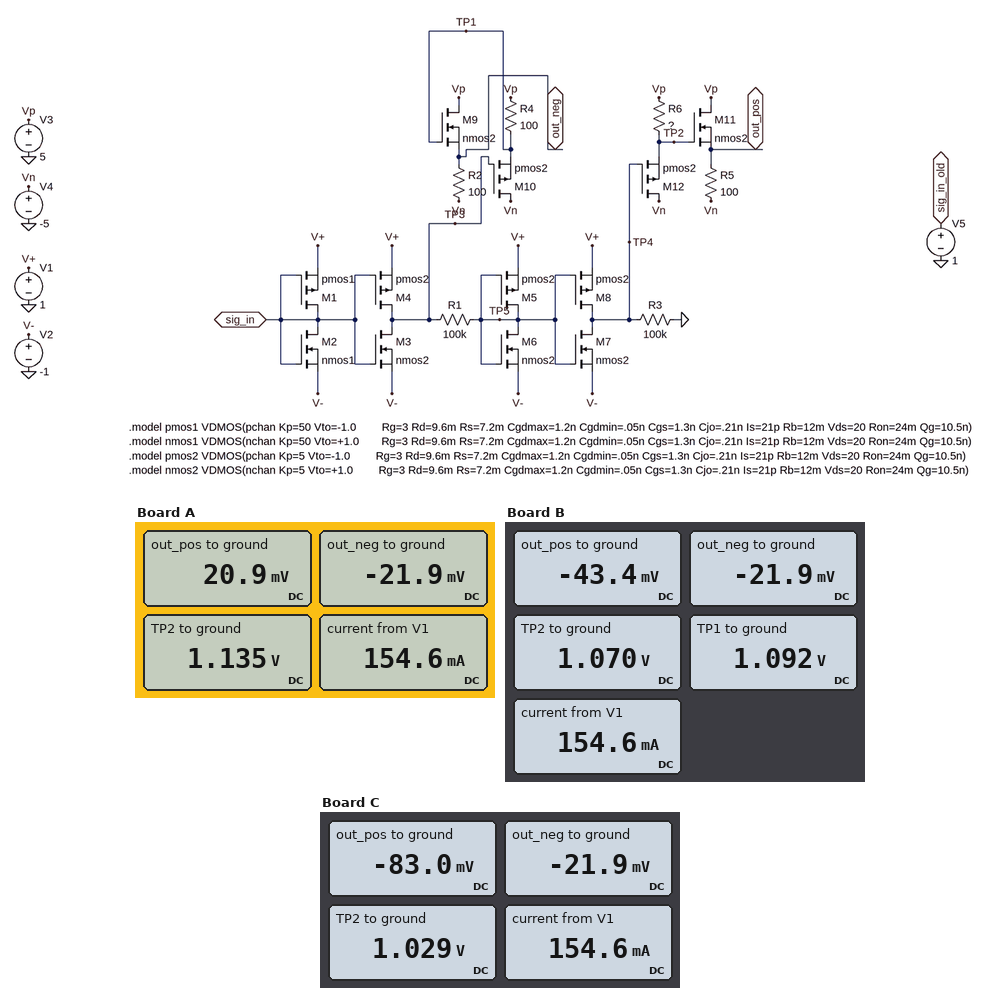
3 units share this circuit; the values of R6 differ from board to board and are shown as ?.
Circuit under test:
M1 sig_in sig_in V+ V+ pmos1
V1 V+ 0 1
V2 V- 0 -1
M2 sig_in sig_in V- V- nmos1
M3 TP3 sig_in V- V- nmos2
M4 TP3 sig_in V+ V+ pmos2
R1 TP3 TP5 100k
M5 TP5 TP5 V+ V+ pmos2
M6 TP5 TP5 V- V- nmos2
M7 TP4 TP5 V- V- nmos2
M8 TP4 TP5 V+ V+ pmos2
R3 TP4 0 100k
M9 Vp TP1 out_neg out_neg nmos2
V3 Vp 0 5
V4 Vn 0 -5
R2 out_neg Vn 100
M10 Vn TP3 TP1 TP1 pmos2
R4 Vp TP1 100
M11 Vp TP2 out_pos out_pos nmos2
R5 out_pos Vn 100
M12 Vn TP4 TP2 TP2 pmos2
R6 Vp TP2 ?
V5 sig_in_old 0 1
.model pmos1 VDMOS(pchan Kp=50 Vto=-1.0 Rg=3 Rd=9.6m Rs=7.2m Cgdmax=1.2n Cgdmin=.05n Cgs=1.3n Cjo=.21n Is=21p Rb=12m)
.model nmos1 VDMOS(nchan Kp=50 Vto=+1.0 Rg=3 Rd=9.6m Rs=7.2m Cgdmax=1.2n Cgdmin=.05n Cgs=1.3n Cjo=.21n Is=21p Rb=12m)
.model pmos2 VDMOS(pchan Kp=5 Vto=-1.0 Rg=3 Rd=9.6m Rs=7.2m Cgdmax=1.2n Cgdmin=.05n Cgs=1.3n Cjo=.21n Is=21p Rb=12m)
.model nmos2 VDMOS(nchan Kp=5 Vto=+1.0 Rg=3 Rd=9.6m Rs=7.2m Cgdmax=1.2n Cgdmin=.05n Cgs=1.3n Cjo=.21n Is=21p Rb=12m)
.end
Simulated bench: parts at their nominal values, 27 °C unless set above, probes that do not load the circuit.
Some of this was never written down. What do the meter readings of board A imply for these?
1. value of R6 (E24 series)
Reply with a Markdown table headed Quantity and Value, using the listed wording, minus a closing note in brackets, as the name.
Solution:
| Quantity | Value |
|---|---|
| value of R6 | 62 Ω |
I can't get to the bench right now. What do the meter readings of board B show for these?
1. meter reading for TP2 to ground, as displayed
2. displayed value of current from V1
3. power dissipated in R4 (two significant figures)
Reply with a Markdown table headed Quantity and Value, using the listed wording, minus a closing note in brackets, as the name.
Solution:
| Quantity | Value |
|---|---|
| meter reading for TP2 to ground, as displayed | 1.070 V |
| displayed value of current from V1 | 154.6 mA |
| power dissipated in R4 | 150 mW |
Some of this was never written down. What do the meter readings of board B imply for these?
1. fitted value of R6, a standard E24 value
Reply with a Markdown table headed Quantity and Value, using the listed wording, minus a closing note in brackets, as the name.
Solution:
| Quantity | Value |
|---|---|
| fitted value of R6, a standard E24 value | 130 Ω |
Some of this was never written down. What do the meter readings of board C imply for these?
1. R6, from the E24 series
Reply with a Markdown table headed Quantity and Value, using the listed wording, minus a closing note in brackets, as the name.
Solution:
| Quantity | Value |
|---|---|
| R6, from the E24 series | 220 Ω |
